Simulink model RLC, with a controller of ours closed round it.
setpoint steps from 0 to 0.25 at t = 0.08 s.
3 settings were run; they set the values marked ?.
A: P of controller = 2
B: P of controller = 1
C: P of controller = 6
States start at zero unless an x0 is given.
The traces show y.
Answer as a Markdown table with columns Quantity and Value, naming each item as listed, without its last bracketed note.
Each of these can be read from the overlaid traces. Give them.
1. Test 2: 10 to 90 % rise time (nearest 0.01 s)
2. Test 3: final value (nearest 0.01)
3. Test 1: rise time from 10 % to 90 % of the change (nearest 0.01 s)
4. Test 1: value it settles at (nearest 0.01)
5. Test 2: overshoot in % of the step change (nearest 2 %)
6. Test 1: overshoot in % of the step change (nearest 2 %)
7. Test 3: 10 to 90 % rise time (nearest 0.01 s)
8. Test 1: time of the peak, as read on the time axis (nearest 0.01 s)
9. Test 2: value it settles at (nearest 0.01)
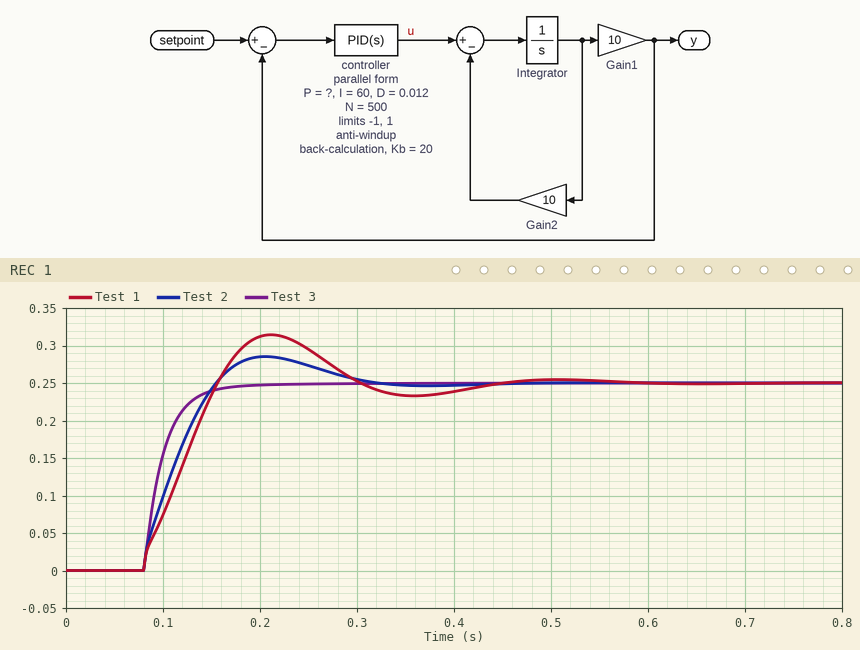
| Quantity | Value |
|---|---|
| Test 2: 10 to 90 % rise time | 0.06 s |
| Test 3: final value | 0.25 |
| Test 1: rise time from 10 % to 90 % of the change | 0.06 s |
| Test 1: value it settles at | 0.25 |
| Test 2: overshoot in % of the step change | 14 % |
| Test 1: overshoot in % of the step change | 26 % |
| Test 3: 10 to 90 % rise time | 0.05 s |
| Test 1: time of the peak, as read on the time axis | 0.21 s |
| Test 2: value it settles at | 0.25 |
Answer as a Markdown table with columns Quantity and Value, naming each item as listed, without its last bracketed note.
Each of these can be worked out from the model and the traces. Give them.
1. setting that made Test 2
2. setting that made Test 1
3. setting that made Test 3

| Quantity | Value |
|---|---|
| setting that made Test 2 | A |
| setting that made Test 1 | B |
| setting that made Test 3 | C |
